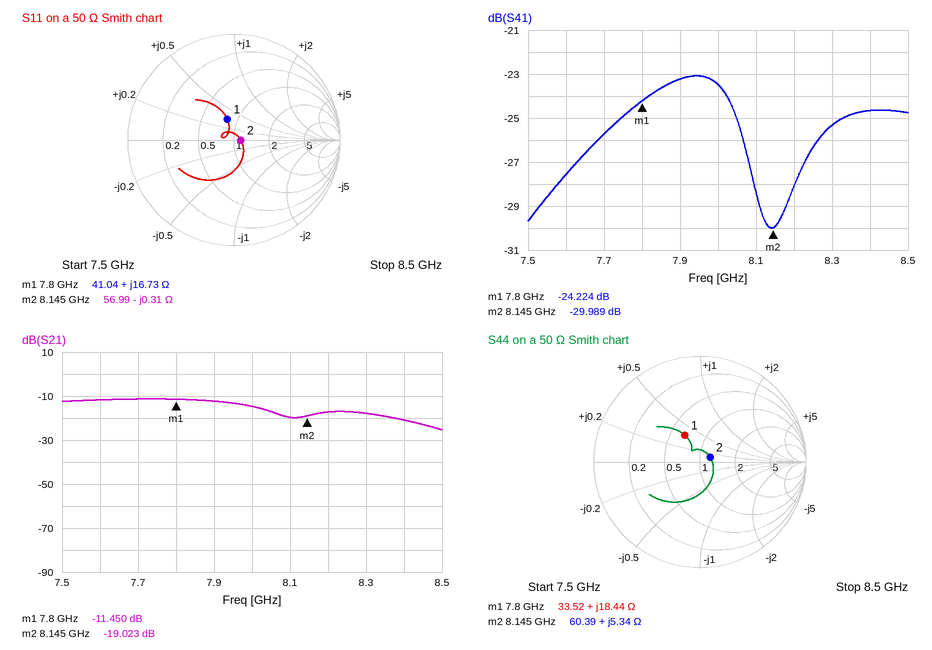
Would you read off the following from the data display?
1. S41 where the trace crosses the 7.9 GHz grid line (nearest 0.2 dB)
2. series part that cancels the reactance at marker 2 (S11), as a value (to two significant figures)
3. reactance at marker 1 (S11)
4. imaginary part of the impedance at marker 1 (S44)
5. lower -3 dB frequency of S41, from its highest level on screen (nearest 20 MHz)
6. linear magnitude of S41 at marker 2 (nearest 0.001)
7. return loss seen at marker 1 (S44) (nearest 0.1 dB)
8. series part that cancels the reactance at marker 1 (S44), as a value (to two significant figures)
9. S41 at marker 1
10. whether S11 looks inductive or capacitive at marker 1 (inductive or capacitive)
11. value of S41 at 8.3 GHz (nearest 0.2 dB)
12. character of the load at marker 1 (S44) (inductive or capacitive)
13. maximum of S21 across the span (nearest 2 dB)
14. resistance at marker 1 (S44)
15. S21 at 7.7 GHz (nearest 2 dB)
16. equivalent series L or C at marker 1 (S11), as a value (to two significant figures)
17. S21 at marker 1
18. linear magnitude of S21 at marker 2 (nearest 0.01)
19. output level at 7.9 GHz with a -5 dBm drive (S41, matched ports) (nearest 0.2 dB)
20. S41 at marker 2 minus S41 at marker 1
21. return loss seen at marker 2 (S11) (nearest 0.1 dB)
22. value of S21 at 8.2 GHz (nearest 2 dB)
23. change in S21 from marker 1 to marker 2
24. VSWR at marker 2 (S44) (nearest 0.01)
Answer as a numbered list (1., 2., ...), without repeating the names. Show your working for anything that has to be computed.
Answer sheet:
1. -23.2 dB
2. L = 0.31 Ω/(2π × 8.145 GHz) ≈ 6.1 pH
3. +16.73 Ω
4. +18.44 Ω
5. 7.68 GHz
6. 10^(-29.989/20) ≈ 0.032
7. 10.8 dB
8. C = 1/(2π × 7.8 GHz × 18.44 Ω) ≈ 1.1 pF
9. -24.224 dB
10. inductive
11. -25.4 dB
12. inductive
13. -12 dB
14. 33.52 Ω
15. -12 dB
16. L = 16.73 Ω/(2π × 7.8 GHz) ≈ 341 pH, so 340 pH to two significant figures
17. -11.450 dB
18. 10^(-19.023/20) ≈ 0.11
19. -5 dBm + (-23.2 dB) = -28.2 dBm
20. -29.989 − (-24.224) = -5.765 dB
21. 23.7 dB
22. -18 dB
23. -19.023 − (-11.45) = -7.573 dB
24. 1.24
